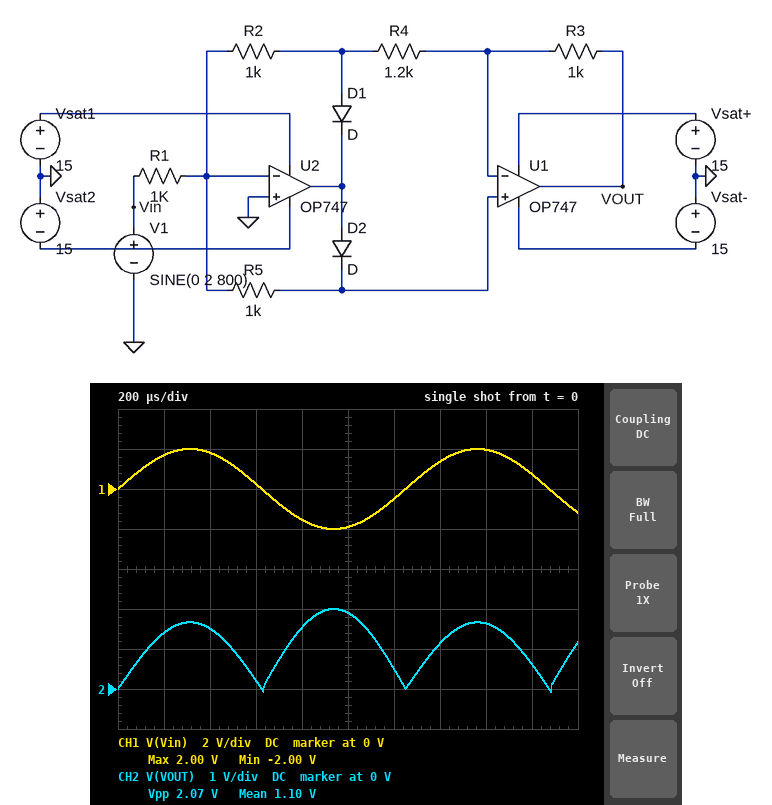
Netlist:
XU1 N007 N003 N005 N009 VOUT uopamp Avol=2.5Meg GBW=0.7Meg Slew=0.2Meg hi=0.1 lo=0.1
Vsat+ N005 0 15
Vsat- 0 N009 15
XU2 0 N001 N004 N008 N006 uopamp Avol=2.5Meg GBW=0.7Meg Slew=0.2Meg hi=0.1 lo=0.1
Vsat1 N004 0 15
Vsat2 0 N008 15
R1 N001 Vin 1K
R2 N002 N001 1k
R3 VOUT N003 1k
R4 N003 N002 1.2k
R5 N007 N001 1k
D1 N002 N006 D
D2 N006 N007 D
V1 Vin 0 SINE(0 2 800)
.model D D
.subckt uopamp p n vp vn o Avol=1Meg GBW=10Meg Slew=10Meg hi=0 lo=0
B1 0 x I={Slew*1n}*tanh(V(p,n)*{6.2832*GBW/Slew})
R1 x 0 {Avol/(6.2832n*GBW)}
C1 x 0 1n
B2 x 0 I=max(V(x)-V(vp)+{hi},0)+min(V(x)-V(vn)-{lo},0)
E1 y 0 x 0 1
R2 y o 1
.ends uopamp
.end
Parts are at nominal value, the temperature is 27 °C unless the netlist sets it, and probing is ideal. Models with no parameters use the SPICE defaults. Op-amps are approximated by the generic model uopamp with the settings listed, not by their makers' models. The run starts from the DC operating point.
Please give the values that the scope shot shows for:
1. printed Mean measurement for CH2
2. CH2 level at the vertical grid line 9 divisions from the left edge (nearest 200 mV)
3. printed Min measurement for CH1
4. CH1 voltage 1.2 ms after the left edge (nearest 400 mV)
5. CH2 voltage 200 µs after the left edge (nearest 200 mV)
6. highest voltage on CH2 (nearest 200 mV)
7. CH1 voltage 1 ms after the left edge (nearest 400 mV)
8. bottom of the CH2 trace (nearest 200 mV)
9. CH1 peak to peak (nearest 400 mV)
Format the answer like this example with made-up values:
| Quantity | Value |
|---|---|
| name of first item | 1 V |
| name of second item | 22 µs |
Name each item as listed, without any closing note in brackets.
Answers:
| Quantity | Value |
|---|---|
| printed Mean measurement for CH2 | 1.10 V |
| CH2 level at the vertical grid line 9 divisions from the left edge | 600 mV |
| printed Min measurement for CH1 | -2.00 V |
| CH1 voltage 1.2 ms after the left edge | -400 mV |
| CH2 voltage 200 µs after the left edge | 1.4 V |
| highest voltage on CH2 | 2.0 V |
| CH1 voltage 1 ms after the left edge | -2.0 V |
| bottom of the CH2 trace | 0 V |
| CH1 peak to peak | 4.0 V |
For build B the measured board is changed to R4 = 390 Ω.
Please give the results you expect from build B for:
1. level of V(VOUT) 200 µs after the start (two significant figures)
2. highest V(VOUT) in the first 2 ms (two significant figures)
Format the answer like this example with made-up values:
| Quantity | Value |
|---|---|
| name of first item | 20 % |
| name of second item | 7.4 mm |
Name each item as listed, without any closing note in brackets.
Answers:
| Quantity | Value |
|---|---|
| level of V(VOUT) 200 µs after the start | 4.3 V |
| highest V(VOUT) in the first 2 ms | 5.1 V |
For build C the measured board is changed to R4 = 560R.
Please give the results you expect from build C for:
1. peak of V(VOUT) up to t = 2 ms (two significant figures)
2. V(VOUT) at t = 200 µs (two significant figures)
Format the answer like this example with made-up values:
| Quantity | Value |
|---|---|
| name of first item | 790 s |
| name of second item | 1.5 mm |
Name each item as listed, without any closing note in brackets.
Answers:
| Quantity | Value |
|---|---|
| peak of V(VOUT) up to t = 2 ms | 3.6 V |
| V(VOUT) at t = 200 µs | 3.0 V |
